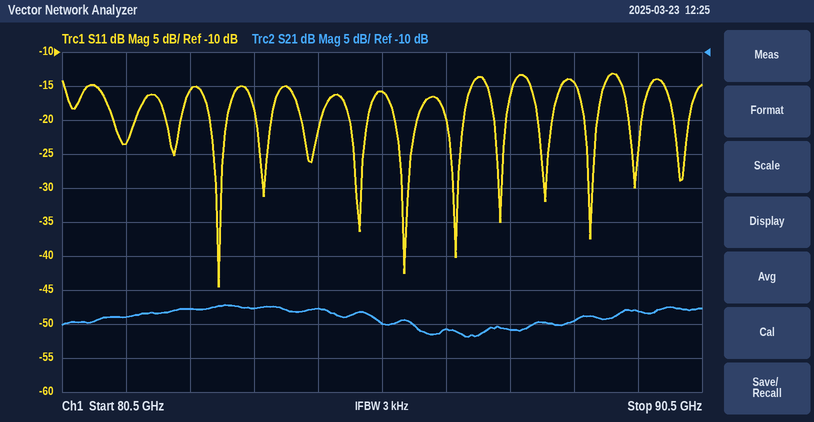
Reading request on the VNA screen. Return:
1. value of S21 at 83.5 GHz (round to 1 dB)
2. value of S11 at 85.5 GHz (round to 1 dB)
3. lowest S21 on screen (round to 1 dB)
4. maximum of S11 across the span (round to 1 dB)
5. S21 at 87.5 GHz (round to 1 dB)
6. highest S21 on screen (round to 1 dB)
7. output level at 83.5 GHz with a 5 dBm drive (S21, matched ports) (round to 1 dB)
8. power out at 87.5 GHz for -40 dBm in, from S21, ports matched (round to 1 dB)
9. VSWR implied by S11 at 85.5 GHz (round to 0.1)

-48 dB
-16 dB
-52 dB
-13 dB
-51 dB
-47 dB
-43 dBm
-91 dBm
1.4
